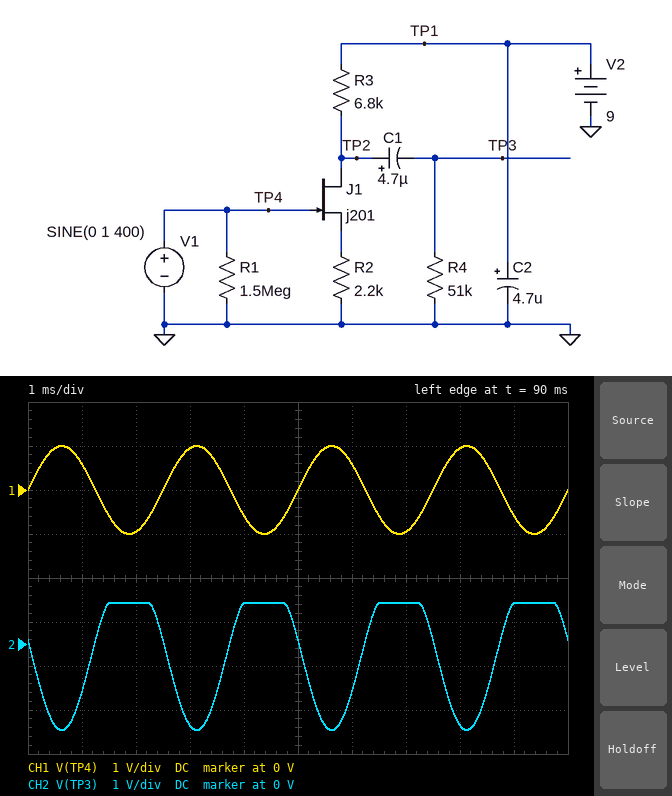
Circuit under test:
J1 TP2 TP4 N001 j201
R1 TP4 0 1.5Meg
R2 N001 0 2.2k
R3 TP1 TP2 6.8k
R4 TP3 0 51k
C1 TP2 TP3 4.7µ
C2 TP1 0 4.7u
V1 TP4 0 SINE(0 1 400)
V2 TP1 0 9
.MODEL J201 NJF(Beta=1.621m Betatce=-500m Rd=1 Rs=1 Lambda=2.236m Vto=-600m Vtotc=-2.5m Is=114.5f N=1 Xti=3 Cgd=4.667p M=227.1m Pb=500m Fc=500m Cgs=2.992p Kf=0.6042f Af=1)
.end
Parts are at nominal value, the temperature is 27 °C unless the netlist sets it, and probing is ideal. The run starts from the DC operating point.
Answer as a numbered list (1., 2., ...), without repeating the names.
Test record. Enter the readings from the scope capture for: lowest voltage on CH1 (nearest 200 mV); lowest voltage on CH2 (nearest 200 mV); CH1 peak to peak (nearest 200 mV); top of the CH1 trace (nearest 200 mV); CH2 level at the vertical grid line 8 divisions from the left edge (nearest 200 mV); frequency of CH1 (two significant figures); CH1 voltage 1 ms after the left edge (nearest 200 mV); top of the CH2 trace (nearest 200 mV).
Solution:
1. -1.0 V
2. -2.0 V
3. 2.0 V
4. 1.0 V
5. -1.8 V
6. 400 Hz
7. 600 mV
8. 1.0 V
